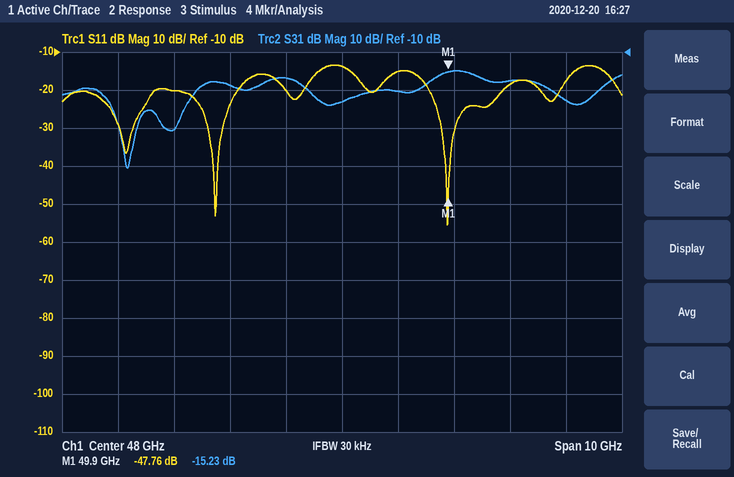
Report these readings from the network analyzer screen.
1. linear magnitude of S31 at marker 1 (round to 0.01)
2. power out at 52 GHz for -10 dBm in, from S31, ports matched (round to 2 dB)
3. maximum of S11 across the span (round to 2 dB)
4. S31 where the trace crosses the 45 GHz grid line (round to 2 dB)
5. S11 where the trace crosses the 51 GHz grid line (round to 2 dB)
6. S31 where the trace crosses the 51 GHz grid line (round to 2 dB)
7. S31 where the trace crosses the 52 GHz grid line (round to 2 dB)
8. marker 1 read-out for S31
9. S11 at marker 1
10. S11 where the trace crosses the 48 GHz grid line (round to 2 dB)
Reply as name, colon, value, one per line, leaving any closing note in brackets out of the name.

linear magnitude of S31 at marker 1: 0.17
power out at 52 GHz for -10 dBm in, from S31, ports matched: -32 dBm
maximum of S11 across the span: -14 dB
S31 where the trace crosses the 45 GHz grid line: -30 dB
S11 where the trace crosses the 51 GHz grid line: -18 dB
S31 where the trace crosses the 51 GHz grid line: -18 dB
S31 where the trace crosses the 52 GHz grid line: -22 dB
marker 1 read-out for S31: -15.23 dB
S11 at marker 1: -47.76 dB
S11 where the trace crosses the 48 GHz grid line: -14 dB
